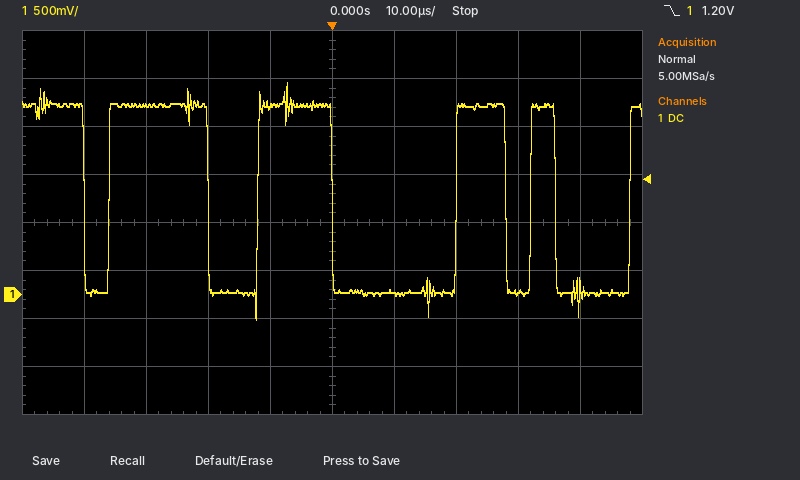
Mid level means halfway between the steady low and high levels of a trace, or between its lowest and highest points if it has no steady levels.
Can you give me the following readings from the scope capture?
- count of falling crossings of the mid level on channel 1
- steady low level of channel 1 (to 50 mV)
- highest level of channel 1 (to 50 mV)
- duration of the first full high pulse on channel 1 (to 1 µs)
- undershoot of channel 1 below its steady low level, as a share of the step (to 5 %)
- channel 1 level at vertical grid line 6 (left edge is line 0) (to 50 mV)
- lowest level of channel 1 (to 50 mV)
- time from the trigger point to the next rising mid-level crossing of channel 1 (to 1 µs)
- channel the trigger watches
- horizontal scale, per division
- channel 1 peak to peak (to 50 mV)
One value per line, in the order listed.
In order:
5
0 mV
2.20 V
16 µs
15 %
0 mV
-250 mV
20 µs
channel 1
10 µs
2.45 V
